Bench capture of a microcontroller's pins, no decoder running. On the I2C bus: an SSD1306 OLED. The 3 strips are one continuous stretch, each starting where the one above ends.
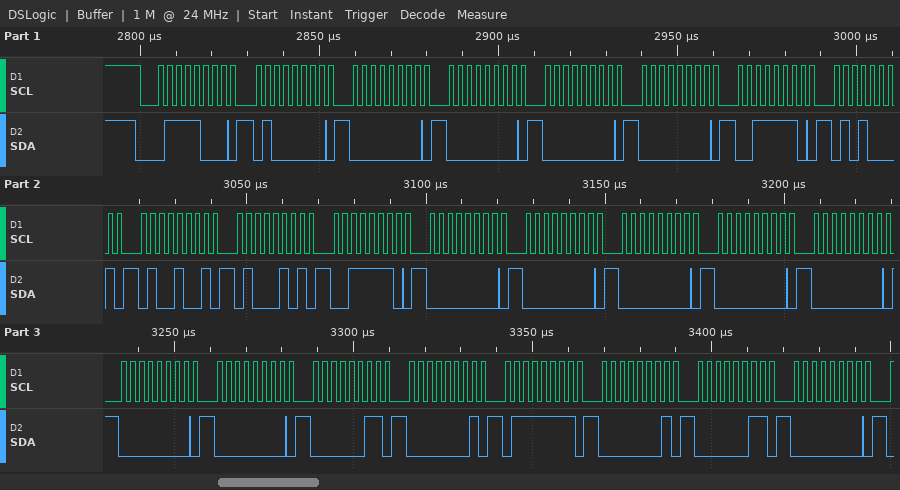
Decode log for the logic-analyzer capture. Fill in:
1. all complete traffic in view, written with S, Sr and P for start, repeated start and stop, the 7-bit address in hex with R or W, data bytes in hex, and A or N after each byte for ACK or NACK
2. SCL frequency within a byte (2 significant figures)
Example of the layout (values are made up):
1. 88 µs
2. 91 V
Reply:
1. S 3CW A 40 A 00 A 00 A 00 A 00 A 3E A 51 A 49 A 45 A 3E A 00 A 00 A 00 A 00 A 00 A 00 A 00 A 03 A 01 A 7F A 01 A 03 A 00 A
2. 400 kHz
